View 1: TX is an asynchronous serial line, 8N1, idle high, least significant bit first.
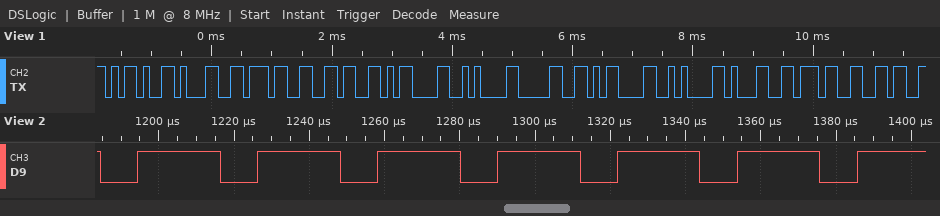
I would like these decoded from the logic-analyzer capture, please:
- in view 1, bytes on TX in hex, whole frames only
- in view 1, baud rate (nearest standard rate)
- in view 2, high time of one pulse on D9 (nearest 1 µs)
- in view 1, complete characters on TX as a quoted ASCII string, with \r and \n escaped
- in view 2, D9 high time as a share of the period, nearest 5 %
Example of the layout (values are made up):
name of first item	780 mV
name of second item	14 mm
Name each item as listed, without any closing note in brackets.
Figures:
in view 1, bytes on TX in hex, whole frames only	2D 31 37 36 0D 0A 30 0D 0A 31 37 36
in view 1, baud rate	9600 baud
in view 2, high time of one pulse on D9	22 µs
in view 1, complete characters on TX as a quoted ASCII string, with \r and \n escaped	"-176\r\n0\r\n176"
in view 2, D9 high time as a share of the period, nearest 5 %	70 %
